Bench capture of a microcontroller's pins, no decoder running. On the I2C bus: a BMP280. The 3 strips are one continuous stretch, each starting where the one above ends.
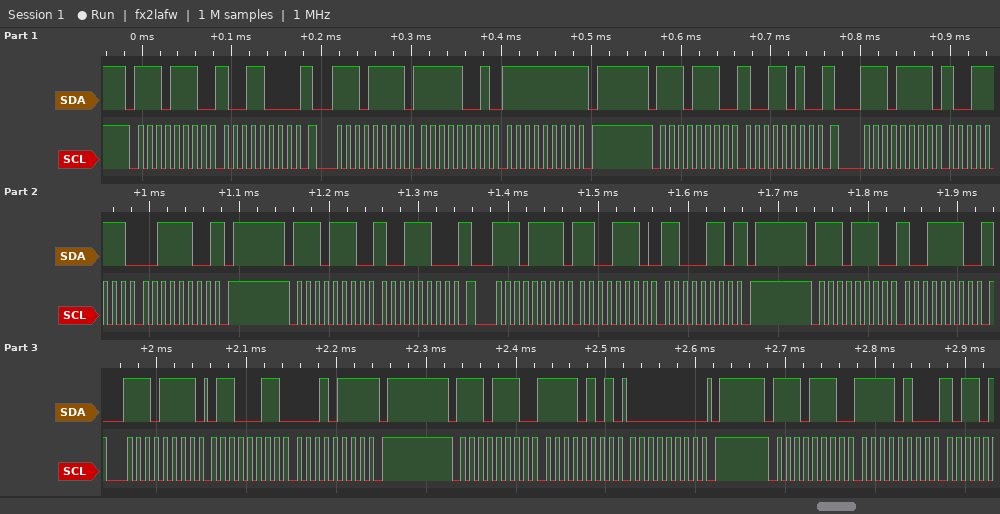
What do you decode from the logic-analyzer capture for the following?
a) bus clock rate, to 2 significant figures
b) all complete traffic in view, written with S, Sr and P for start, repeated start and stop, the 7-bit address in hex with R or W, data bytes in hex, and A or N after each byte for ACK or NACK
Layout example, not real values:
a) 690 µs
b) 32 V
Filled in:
a) 100 kHz
b) S 77W A 98 A Sr 77R A F9 A FF N P S 77W A 9A A Sr 77R A 9F A 3C N P S 77W A 9C A Sr 77R A CE A C6 N P S 77W A 9E A Sr 77R A 63 A 17 N P S 77W A F5 A 00 A P S 77W A F4 A
